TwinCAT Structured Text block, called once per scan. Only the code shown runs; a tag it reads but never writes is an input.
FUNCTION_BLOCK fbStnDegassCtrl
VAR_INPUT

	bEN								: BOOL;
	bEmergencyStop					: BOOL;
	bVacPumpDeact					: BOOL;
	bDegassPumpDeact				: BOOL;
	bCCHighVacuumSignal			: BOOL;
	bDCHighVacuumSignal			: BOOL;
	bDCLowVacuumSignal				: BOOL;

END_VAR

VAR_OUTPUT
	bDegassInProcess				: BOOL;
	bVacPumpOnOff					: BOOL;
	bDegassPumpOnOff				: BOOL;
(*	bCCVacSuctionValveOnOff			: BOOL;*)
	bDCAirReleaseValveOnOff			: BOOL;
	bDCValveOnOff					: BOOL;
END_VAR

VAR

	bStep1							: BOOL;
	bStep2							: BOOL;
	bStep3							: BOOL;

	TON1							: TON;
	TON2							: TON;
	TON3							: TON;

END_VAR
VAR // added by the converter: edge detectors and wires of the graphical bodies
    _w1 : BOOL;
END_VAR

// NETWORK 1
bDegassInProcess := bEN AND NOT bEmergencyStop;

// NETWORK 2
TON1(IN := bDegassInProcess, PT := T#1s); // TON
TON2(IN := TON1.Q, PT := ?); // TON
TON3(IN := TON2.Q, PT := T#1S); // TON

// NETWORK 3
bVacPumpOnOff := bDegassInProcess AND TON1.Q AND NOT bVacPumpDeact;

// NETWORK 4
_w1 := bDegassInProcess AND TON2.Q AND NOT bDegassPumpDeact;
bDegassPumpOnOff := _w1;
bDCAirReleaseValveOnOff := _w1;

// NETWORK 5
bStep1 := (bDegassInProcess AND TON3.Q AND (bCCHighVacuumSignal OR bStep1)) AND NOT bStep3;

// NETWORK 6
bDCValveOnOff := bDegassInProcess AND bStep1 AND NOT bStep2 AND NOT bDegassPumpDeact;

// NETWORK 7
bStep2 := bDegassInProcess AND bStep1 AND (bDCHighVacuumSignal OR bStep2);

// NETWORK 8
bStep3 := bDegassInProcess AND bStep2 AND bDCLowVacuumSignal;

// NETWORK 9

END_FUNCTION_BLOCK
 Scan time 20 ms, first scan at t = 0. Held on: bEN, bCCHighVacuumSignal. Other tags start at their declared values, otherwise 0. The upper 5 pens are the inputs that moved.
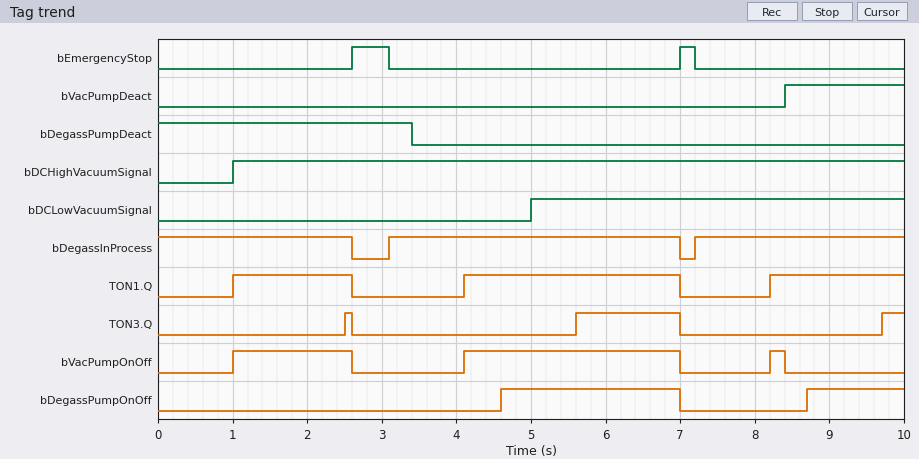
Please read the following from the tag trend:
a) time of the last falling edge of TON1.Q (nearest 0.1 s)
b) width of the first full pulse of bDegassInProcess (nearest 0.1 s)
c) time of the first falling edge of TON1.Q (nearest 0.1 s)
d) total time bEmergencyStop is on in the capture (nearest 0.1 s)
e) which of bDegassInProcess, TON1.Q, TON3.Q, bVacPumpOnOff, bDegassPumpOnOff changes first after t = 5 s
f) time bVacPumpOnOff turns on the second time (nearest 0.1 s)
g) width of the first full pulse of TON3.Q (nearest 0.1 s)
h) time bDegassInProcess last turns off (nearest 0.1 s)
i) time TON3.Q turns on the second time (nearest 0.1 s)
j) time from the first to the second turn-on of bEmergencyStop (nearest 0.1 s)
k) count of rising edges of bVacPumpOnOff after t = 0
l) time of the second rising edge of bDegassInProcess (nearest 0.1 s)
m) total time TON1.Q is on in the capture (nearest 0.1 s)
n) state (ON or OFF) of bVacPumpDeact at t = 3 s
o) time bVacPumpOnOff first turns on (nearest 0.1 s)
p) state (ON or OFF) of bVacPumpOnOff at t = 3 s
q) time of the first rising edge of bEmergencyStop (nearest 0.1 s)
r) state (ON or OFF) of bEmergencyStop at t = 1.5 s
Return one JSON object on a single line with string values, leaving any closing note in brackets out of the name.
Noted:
{"time of the last falling edge of TON1.Q": "7.0 s", "width of the first full pulse of bDegassInProcess": "3.9 s", "time of the first falling edge of TON1.Q": "2.6 s", "total time bEmergencyStop is on in the capture": "0.7 s", "which of bDegassInProcess, TON1.Q, TON3.Q, bVacPumpOnOff, bDegassPumpOnOff changes first after t = 5 s": "TON3.Q", "time bVacPumpOnOff turns on the second time": "4.1 s", "width of the first full pulse of TON3.Q": "0.1 s", "time bDegassInProcess last turns off": "7.0 s", "time TON3.Q turns on the second time": "5.6 s", "time from the first to the second turn-on of bEmergencyStop": "4.4 s", "count of rising edges of bVacPumpOnOff after t = 0": "3", "time of the second rising edge of bDegassInProcess": "7.2 s", "total time TON1.Q is on in the capture": "6.3 s", "state (ON or OFF) of bVacPumpDeact at t = 3 s": "OFF", "time bVacPumpOnOff first turns on": "1.0 s", "state (ON or OFF) of bVacPumpOnOff at t = 3 s": "OFF", "time of the first rising edge of bEmergencyStop": "2.6 s", "state (ON or OFF) of bEmergencyStop at t = 1.5 s": "OFF"}
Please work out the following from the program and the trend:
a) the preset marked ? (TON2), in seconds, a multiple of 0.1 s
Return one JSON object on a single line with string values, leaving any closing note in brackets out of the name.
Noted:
{"the preset marked ? (TON2), in seconds, a multiple of 0.1 s": "0.5 s"}
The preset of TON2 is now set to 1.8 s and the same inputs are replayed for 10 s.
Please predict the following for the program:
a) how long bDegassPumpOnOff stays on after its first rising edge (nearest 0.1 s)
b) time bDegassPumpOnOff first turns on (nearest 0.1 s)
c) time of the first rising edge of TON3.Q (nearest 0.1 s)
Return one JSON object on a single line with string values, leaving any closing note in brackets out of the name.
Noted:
{"how long bDegassPumpOnOff stays on after its first rising edge": "1.1 s", "time bDegassPumpOnOff first turns on": "5.9 s", "time of the first rising edge of TON3.Q": "6.9 s"}
